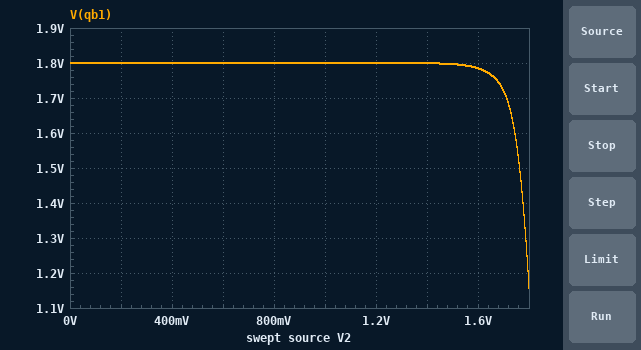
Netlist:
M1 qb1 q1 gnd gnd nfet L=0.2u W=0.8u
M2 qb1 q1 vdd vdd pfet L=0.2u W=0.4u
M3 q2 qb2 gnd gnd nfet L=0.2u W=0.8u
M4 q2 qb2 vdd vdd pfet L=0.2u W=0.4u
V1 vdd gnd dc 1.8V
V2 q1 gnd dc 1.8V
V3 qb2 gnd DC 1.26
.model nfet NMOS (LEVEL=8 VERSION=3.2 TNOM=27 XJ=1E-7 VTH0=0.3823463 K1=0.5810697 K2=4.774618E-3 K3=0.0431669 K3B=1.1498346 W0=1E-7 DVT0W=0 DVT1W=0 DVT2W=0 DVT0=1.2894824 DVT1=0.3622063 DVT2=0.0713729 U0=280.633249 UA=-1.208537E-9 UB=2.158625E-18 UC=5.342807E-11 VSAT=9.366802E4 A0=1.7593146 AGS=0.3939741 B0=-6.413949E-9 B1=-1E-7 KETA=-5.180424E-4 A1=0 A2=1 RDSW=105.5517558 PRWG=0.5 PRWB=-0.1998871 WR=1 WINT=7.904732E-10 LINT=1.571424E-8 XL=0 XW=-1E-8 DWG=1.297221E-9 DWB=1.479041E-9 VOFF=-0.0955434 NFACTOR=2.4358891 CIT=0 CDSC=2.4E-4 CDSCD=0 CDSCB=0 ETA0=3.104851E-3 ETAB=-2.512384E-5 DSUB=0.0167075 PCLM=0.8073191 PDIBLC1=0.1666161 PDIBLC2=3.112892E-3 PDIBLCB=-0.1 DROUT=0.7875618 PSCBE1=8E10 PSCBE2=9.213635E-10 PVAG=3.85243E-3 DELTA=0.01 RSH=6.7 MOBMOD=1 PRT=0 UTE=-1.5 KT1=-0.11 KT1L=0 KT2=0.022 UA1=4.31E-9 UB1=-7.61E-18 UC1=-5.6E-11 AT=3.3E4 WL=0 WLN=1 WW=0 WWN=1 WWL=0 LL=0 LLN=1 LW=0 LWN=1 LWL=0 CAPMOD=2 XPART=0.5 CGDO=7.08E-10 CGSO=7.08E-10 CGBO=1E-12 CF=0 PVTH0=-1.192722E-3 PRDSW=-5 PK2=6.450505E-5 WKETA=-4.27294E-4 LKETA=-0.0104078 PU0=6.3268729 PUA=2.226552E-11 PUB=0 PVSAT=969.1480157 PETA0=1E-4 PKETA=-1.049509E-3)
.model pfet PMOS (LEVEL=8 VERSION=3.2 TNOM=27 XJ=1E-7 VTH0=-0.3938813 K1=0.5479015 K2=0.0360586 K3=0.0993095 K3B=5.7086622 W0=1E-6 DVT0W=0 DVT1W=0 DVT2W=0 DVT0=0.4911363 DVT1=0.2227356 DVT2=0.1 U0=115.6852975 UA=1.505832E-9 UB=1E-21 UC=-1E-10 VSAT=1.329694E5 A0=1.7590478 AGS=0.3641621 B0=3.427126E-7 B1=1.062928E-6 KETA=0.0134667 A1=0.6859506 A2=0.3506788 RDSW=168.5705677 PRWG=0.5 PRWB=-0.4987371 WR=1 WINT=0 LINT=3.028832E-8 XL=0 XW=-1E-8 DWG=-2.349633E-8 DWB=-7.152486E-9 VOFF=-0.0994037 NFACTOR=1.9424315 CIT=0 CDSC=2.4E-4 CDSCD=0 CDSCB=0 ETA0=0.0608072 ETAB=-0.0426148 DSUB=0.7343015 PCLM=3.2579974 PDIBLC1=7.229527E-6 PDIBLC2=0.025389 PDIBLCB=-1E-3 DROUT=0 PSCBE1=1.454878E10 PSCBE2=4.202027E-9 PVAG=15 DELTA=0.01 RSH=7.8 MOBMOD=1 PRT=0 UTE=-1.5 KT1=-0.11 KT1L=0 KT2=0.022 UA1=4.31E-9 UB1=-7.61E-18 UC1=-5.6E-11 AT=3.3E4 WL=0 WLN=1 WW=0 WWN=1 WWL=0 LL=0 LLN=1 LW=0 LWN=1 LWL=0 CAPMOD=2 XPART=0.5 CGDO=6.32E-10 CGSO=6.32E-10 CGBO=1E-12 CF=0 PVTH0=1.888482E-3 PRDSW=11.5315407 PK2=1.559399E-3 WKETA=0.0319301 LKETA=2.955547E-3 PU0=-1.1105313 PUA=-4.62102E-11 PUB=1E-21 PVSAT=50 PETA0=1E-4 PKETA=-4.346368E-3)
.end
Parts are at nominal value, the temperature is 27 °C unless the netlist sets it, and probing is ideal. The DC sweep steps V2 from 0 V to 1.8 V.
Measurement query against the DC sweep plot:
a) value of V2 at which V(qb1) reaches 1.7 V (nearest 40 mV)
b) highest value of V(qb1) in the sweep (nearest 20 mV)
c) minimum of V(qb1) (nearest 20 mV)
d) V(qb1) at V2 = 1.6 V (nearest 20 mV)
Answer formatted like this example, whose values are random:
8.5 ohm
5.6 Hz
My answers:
1.72 V
1.80 V
1.16 V
1.78 V
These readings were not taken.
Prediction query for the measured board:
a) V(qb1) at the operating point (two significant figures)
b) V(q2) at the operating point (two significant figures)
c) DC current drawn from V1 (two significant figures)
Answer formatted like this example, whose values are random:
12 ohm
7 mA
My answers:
1.2 V
1.8 V
1.5 mA
